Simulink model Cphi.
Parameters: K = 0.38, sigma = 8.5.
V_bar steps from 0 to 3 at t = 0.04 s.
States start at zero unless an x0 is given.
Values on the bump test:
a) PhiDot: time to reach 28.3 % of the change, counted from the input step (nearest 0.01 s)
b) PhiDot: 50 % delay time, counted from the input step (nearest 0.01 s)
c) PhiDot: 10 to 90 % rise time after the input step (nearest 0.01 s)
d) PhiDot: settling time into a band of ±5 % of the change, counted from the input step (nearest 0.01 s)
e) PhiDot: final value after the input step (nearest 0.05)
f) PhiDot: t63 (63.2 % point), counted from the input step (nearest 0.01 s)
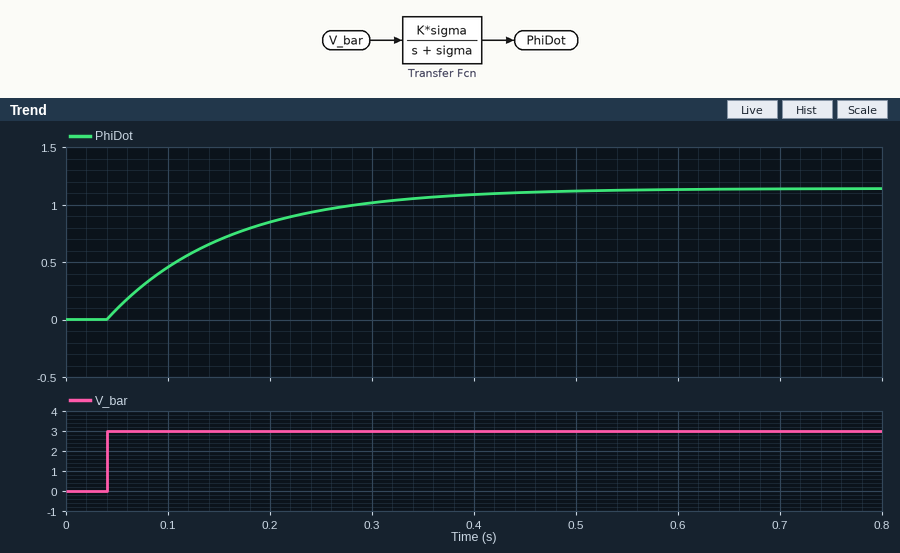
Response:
0.04 s
0.08 s
0.26 s
0.35 s
1.15
0.12 s
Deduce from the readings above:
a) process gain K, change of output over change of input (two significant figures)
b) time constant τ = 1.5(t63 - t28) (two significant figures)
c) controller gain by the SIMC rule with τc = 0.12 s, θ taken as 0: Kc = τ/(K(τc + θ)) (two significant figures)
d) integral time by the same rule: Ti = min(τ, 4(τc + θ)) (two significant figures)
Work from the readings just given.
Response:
0.38
0.12 s
2.6
0.12 s
